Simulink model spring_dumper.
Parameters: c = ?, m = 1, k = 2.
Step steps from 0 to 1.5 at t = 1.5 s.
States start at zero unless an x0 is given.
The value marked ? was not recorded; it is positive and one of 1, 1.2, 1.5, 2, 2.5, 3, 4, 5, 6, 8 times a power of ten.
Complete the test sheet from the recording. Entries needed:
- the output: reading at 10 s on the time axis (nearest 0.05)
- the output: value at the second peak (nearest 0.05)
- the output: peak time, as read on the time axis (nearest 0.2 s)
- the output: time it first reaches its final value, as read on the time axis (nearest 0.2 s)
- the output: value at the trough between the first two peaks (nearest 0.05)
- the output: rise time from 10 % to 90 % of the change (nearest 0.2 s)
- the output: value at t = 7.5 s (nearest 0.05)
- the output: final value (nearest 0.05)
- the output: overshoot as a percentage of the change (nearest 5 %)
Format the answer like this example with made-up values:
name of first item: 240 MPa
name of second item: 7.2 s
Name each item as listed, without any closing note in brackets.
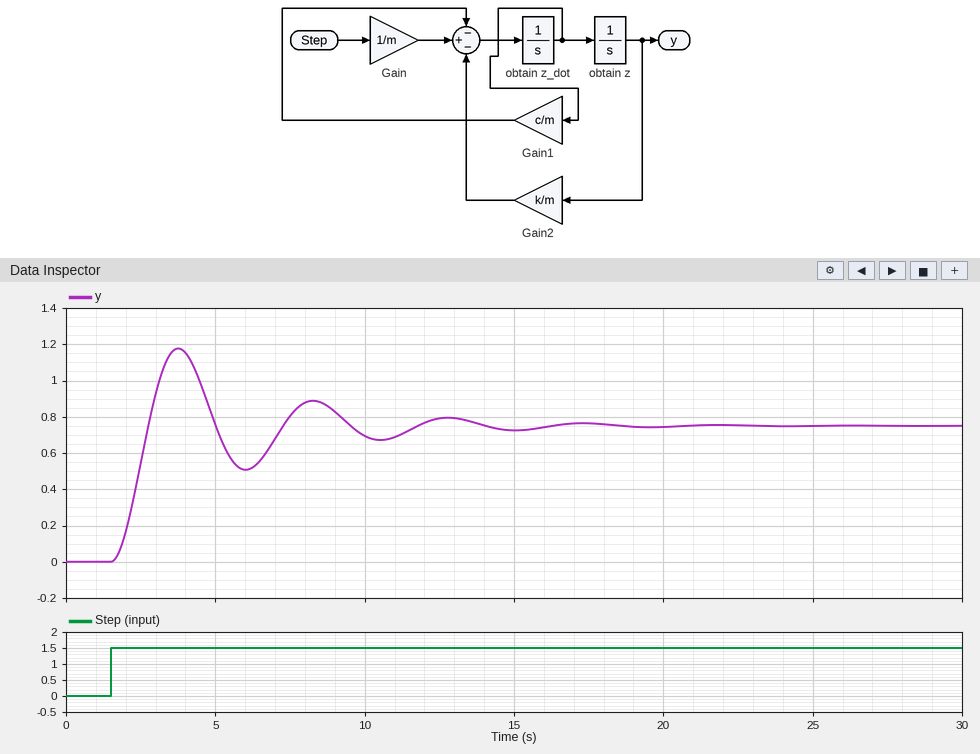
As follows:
the output: reading at 10 s on the time axis: 0.70
the output: value at the second peak: 0.90
the output: peak time, as read on the time axis: 3.8 s
the output: time it first reaches its final value, as read on the time axis: 2.8 s
the output: value at the trough between the first two peaks: 0.50
the output: rise time from 10 % to 90 % of the change: 0.8 s
the output: value at t = 7.5 s: 0.80
the output: final value: 0.75
the output: overshoot as a percentage of the change: 55 %
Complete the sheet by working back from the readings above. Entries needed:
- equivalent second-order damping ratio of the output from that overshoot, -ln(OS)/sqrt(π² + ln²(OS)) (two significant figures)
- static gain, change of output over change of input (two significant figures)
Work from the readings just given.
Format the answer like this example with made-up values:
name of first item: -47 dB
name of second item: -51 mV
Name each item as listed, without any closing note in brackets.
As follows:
equivalent second-order damping ratio of the output from that overshoot, -ln(OS)/sqrt(π² + ln²(OS)): 0.19
static gain, change of output over change of input: 0.50
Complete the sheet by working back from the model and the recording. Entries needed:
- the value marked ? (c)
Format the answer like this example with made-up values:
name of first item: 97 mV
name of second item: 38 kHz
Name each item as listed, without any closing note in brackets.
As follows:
the value marked ?: 0.5
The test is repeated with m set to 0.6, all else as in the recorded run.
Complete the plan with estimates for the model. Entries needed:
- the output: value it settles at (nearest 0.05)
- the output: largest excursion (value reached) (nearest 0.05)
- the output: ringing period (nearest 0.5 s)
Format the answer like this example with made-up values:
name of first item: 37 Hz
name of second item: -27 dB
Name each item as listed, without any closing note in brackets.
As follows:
the output: value it settles at: 0.75
the output: largest excursion (value reached): 1.10
the output: ringing period: 3.5 s
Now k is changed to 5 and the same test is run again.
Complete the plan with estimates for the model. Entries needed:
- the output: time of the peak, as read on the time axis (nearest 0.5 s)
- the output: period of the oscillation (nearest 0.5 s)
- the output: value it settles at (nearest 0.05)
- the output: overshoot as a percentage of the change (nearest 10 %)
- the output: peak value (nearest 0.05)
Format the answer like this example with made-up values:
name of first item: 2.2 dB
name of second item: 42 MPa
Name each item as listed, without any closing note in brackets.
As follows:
the output: time of the peak, as read on the time axis: 3.0 s
the output: period of the oscillation: 3.0 s
the output: value it settles at: 0.30
the output: overshoot as a percentage of the change: 70 %
the output: peak value: 0.50
